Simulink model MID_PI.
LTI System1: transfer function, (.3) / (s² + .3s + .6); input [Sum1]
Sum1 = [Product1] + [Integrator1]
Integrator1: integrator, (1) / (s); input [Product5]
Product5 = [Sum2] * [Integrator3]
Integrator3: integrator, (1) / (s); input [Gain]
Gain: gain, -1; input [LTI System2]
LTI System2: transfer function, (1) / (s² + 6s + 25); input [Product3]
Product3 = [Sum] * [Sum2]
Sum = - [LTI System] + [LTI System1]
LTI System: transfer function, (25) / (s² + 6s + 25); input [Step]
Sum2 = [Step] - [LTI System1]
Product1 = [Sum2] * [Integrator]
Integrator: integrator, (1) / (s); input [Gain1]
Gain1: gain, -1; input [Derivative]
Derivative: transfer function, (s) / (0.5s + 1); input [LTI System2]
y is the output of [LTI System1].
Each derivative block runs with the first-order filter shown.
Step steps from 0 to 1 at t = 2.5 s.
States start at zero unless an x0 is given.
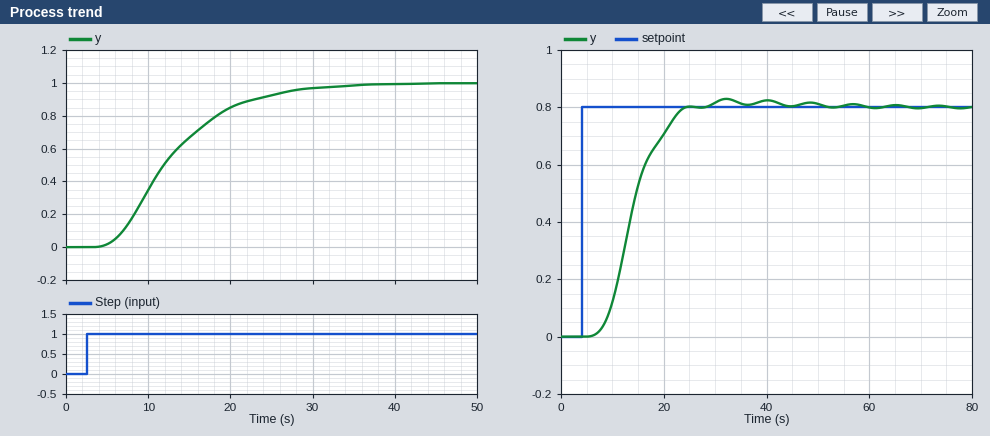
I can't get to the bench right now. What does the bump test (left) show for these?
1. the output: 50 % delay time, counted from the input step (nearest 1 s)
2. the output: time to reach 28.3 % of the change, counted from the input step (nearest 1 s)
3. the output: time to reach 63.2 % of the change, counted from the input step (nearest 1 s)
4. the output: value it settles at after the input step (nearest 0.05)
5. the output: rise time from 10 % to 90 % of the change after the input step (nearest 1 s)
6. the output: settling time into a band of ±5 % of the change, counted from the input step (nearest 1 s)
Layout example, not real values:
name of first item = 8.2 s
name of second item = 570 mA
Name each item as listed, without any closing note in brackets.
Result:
the output: 50 % delay time, counted from the input step = 9 s
the output: time to reach 28.3 % of the change, counted from the input step = 7 s
the output: time to reach 63.2 % of the change, counted from the input step = 12 s
the output: value it settles at after the input step = 1.00
the output: rise time from 10 % to 90 % of the change after the input step = 16 s
the output: settling time into a band of ±5 % of the change, counted from the input step = 25 s
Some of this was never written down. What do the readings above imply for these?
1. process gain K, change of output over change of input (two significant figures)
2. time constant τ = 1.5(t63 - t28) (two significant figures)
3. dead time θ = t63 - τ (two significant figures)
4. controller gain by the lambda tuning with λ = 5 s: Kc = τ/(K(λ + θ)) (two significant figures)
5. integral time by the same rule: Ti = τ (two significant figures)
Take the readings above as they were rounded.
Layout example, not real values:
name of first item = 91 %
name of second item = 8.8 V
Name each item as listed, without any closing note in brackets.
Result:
process gain K, change of output over change of input = 1.0
time constant τ = 1.5(t63 - t28) = 7.5 s
dead time θ = t63 - τ = 4.5 s
controller gain by the lambda tuning with λ = 5 s: Kc = τ/(K(λ + θ)) = 0.79
integral time by the same rule: Ti = τ = 7.5 s
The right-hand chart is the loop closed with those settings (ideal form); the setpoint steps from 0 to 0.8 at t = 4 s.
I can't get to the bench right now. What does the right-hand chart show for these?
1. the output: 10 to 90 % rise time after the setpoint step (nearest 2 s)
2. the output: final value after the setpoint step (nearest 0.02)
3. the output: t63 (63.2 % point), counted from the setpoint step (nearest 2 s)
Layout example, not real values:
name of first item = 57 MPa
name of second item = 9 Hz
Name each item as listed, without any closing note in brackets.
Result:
the output: 10 to 90 % rise time after the setpoint step = 12 s
the output: final value after the setpoint step = 0.80
the output: t63 (63.2 % point), counted from the setpoint step = 10 s
